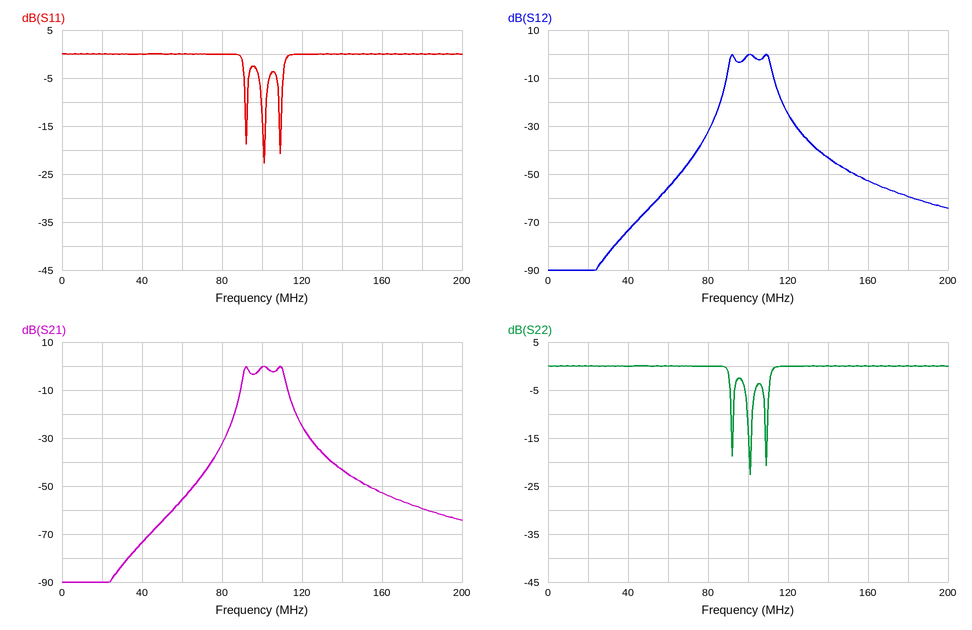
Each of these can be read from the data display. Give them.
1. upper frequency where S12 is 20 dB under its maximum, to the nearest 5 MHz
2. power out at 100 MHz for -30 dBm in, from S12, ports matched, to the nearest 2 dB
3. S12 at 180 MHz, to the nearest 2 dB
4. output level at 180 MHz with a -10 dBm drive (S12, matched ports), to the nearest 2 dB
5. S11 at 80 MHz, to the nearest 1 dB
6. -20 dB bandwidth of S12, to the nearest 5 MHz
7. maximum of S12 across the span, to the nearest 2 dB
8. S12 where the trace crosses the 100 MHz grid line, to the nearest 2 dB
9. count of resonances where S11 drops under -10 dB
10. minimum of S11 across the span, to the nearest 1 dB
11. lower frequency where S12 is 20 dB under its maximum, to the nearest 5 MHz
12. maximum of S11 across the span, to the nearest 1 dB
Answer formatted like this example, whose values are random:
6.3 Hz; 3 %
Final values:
115 MHz; -30 dBm; -60 dB; -70 dBm; 0 dB; 30 MHz; 0 dB; 0 dB; 3; -23 dB; 85 MHz; 0 dB
